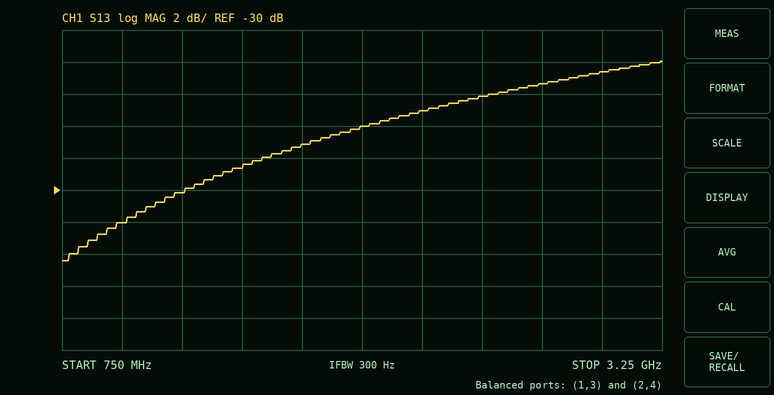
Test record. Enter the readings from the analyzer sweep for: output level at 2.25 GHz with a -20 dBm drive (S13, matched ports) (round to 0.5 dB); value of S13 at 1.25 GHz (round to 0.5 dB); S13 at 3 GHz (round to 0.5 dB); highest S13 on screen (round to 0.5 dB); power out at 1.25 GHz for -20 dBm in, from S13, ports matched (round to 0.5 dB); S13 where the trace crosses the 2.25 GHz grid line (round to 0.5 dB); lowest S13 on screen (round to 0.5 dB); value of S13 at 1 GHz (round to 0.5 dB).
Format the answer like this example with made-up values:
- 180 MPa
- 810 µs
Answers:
- -45.0 dBm
- -30.0 dB
- -22.5 dB
- -22.0 dB
- -50.0 dBm
- -25.0 dB
- -34.5 dB
- -32.0 dB
